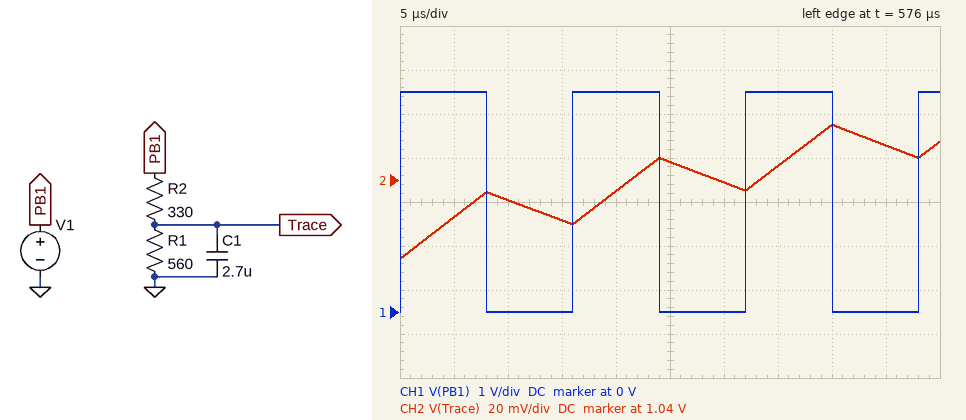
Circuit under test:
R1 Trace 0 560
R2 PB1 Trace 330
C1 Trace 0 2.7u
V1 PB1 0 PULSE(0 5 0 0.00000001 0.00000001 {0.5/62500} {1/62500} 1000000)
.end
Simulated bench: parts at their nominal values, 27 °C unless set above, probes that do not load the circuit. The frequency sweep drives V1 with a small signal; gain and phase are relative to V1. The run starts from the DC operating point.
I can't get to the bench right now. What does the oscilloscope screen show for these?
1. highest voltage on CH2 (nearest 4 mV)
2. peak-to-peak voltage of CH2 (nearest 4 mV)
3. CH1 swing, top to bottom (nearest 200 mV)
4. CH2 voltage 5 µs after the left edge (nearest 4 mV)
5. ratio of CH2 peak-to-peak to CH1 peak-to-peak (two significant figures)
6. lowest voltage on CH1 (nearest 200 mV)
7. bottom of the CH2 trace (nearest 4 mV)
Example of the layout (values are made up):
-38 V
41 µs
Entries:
1.064 V
60 mV
5.0 V
1.024 V
0.012
0 V
1.004 V
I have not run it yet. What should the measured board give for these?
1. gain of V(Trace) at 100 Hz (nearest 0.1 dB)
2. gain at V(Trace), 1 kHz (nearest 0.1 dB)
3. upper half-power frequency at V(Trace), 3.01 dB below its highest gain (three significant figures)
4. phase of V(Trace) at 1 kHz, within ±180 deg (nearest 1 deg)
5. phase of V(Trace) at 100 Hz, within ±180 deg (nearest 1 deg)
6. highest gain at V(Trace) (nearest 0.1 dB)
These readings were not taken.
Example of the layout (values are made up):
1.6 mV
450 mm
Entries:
-4.5 dB
-15.3 dB
284 Hz
-74 deg
-19 deg
-4.0 dB
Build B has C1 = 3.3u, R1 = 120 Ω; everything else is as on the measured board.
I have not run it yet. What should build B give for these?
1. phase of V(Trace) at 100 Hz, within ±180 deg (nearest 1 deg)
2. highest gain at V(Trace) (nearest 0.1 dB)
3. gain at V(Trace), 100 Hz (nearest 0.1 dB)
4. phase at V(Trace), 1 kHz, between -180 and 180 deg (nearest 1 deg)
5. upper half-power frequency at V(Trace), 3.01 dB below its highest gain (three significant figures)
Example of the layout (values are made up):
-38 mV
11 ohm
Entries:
-10 deg
-11.5 dB
-11.6 dB
-61 deg
548 Hz
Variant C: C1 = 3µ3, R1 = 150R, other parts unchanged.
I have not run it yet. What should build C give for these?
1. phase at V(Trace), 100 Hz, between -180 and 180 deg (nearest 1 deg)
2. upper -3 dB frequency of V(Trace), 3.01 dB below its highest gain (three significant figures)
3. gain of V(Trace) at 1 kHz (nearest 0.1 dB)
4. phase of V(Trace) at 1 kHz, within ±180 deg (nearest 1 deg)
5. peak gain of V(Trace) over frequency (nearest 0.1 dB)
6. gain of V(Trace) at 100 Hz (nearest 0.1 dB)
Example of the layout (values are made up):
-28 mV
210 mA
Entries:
-12 deg
468 Hz
-17.6 dB
-65 deg
-10.1 dB
-10.3 dB
